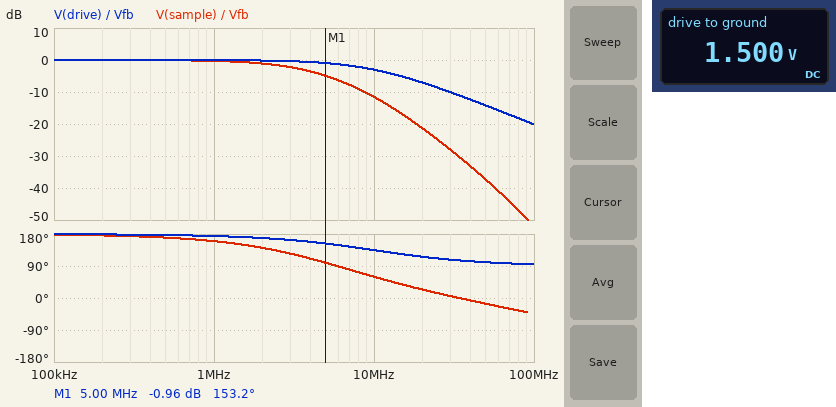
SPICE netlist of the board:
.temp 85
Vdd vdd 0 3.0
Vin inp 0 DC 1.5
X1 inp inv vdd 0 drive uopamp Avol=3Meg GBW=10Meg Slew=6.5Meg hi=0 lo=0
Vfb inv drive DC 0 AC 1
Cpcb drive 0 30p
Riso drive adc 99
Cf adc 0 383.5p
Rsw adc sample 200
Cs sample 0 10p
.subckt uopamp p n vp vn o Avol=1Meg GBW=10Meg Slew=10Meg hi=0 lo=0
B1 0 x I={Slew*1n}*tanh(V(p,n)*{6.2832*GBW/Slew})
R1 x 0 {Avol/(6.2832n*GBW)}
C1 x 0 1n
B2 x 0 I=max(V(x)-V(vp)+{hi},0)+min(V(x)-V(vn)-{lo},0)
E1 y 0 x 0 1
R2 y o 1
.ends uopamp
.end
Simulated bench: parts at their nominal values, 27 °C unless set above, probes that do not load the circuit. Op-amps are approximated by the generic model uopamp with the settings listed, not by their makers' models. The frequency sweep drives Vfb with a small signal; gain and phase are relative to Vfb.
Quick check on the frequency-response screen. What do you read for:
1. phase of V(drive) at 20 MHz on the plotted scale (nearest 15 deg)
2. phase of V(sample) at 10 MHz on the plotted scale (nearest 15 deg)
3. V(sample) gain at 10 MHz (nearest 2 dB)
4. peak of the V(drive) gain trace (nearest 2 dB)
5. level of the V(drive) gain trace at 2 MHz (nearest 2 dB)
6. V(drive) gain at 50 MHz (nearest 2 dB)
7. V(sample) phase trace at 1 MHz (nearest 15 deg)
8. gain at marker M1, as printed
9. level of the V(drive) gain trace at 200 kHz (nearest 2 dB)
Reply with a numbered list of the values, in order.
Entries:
1. 120 deg
2. 60 deg
3. -12 dB
4. 0 dB
5. 0 dB
6. -14 dB
7. 165 deg
8. -0.96 dB
9. 0 dB
